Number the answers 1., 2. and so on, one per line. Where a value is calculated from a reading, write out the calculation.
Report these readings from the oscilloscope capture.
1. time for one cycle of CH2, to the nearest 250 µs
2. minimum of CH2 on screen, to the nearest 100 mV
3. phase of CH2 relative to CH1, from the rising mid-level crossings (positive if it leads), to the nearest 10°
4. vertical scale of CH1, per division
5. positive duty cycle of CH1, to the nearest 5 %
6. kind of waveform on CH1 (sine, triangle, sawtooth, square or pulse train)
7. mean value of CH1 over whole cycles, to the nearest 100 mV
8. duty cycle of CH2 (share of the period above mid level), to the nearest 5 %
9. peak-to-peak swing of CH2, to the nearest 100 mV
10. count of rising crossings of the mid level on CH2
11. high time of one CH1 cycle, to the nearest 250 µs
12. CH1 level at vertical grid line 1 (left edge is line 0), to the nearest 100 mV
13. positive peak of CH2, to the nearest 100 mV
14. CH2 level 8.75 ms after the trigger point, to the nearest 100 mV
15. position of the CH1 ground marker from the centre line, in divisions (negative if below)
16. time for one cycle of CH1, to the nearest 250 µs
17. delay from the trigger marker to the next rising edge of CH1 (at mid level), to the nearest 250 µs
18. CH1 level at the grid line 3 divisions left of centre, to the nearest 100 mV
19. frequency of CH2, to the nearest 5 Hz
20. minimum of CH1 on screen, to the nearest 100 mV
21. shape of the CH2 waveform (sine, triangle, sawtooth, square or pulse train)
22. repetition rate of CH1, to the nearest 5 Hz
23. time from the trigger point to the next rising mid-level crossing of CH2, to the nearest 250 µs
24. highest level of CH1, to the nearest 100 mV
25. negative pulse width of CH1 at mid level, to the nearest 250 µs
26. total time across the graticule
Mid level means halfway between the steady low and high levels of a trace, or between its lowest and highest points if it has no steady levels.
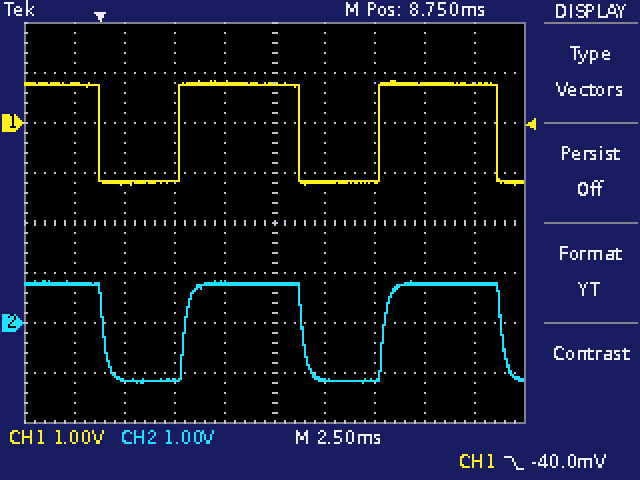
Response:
1. 10.00 ms
2. -1.2 V
3. −360° × (+250 µs) / 10.00 ms ≈ -9.00°, so -10° to the nearest 10°
4. 1 V
5. 6.00 ms / 10.00 ms ≈ 60 %
6. pulse train
7. -1.2 V + 0.6 × (800 mV − (-1.2 V)) ≈ 0.0 V
8. 6.00 ms / 10.00 ms ≈ 60 %
9. 800 mV − (-1.2 V) = 2.0 V
10. 2
11. 6.00 ms
12. 800 mV
13. 800 mV
14. 800 mV
15. +2.0 div
16. 10.00 ms
17. 4.00 ms
18. -1.2 V
19. 1 / 10.00 ms ≈ 100 Hz
20. -1.2 V
21. pulse train
22. 1 / 10.00 ms ≈ 100 Hz
23. 4.25 ms
24. 800 mV
25. 4.00 ms
26. 25 ms
